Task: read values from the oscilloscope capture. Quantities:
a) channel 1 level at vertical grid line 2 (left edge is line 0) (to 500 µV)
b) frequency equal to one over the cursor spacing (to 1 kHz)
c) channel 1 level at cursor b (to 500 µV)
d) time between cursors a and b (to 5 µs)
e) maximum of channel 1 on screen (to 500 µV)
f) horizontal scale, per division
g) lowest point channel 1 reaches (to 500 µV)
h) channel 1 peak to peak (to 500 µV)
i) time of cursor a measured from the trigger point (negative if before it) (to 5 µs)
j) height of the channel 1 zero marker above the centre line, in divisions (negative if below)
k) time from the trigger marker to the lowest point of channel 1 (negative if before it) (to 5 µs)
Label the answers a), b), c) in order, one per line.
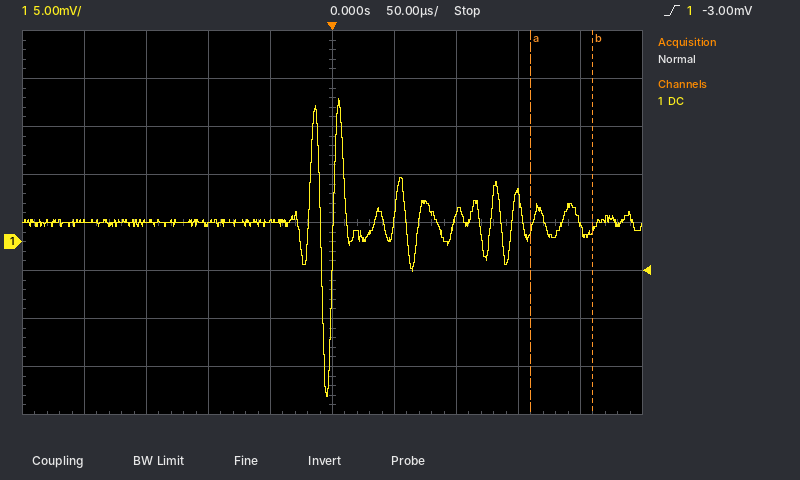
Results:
a) 2.0 mV
b) 20 kHz
c) 1.0 mV
d) 50 µs
e) 15.0 mV
f) 50 µs
g) -16.0 mV
h) 31.0 mV
i) +160 µs
j) -0.4 div
k) -5 µs
